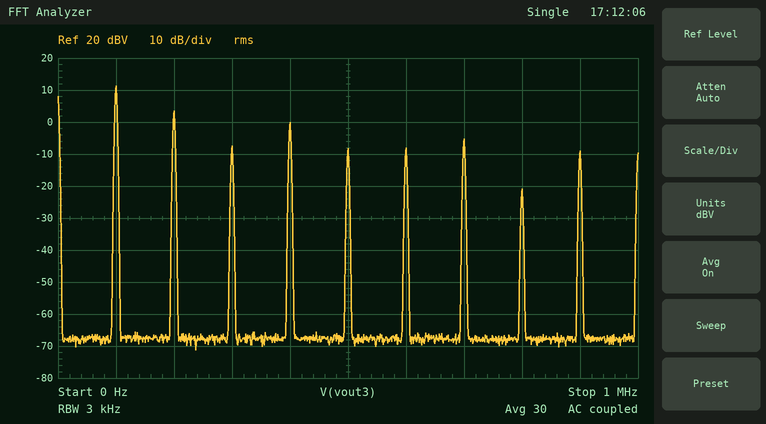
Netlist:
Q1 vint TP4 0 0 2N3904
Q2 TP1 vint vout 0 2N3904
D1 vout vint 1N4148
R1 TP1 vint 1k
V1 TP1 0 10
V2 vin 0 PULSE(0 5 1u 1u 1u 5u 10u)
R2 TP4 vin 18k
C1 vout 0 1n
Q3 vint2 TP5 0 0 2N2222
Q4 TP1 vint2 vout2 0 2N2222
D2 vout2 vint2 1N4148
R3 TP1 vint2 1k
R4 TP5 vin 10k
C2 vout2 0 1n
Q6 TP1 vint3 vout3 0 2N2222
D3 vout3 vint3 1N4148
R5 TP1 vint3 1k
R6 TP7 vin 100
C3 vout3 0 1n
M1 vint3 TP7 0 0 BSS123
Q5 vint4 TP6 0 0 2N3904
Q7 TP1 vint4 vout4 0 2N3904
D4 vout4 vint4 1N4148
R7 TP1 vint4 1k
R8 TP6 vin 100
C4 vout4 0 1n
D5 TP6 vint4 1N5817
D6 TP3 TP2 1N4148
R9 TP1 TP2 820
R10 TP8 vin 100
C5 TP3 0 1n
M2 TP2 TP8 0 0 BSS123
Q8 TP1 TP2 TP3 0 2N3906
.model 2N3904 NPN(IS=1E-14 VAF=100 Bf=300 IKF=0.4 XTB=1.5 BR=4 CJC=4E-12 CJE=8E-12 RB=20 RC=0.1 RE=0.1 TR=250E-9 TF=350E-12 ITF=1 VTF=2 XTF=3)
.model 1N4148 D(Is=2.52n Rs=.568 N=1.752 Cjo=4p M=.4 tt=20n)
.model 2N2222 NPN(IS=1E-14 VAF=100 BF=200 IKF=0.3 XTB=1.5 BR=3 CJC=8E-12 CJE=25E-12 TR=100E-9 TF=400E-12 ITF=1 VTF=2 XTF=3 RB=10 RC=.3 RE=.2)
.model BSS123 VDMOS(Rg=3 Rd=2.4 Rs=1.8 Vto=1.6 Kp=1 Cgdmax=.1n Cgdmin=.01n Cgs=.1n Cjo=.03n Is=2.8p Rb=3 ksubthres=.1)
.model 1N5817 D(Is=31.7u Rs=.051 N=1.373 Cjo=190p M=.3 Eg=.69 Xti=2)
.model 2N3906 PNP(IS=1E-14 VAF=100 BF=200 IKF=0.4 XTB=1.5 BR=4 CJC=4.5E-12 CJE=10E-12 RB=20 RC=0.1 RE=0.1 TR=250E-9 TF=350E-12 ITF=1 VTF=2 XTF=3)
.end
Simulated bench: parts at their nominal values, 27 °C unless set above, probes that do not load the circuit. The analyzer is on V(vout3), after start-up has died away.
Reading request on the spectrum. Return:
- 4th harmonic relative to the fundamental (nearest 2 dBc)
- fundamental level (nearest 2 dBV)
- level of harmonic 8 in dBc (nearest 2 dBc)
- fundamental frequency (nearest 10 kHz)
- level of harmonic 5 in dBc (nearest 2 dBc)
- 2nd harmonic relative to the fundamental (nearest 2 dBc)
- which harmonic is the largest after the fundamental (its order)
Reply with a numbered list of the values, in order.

1. -12 dBc
2. 12 dBV
3. -32 dBc
4. 100 kHz
5. -20 dBc
6. -8 dBc
7. 2
